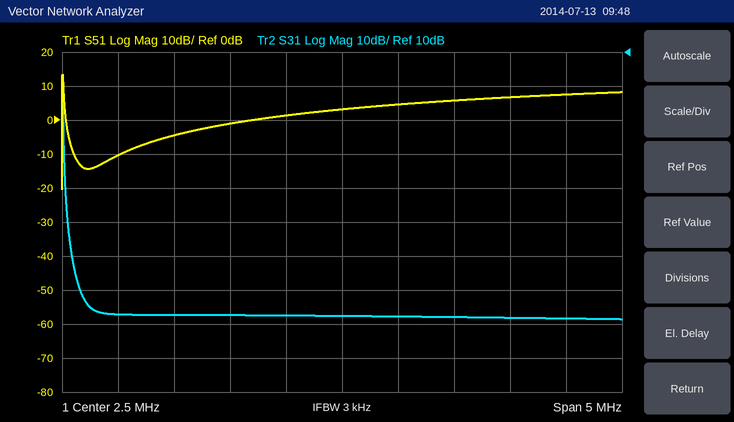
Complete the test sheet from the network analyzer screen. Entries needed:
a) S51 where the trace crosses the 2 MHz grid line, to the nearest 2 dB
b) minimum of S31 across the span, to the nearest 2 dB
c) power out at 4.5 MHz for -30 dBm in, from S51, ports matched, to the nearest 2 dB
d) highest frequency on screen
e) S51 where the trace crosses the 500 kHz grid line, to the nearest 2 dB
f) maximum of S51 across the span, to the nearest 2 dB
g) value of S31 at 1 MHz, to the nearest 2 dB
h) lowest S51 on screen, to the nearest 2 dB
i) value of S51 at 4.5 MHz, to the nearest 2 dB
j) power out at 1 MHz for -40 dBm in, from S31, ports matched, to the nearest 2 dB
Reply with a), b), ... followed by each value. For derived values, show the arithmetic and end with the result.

a) 2 dB
b) -68 dB
c) -30 dBm + (8 dB) = -22 dBm
d) 5 MHz
e) -10 dB
f) 14 dB
g) -68 dB
h) -20 dB
i) 8 dB
j) -40 dBm + (-68 dB) = -108 dBm
